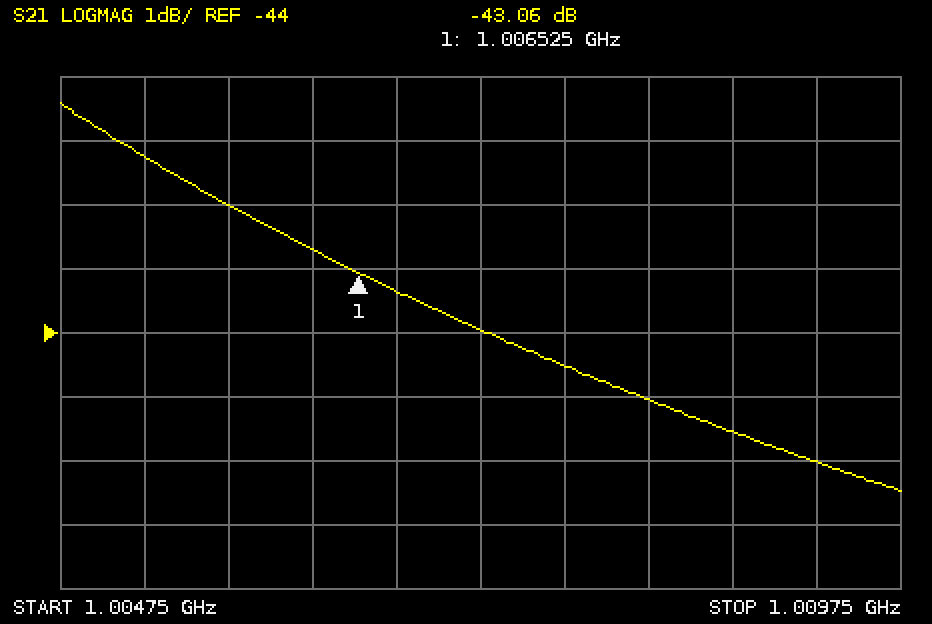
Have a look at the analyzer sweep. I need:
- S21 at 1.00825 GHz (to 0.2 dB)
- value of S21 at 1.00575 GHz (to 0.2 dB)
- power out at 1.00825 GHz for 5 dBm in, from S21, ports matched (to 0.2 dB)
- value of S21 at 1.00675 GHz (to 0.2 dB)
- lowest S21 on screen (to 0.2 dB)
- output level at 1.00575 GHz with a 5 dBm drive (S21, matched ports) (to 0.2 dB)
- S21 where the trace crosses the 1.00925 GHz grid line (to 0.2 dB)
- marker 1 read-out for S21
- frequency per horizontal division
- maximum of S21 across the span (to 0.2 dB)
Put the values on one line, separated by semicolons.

-45.0 dB; -42.0 dB; -40.0 dBm; -43.4 dB; -46.4 dB; -37.0 dBm; -46.0 dB; -43.06 dB; 500 kHz; -40.4 dB
